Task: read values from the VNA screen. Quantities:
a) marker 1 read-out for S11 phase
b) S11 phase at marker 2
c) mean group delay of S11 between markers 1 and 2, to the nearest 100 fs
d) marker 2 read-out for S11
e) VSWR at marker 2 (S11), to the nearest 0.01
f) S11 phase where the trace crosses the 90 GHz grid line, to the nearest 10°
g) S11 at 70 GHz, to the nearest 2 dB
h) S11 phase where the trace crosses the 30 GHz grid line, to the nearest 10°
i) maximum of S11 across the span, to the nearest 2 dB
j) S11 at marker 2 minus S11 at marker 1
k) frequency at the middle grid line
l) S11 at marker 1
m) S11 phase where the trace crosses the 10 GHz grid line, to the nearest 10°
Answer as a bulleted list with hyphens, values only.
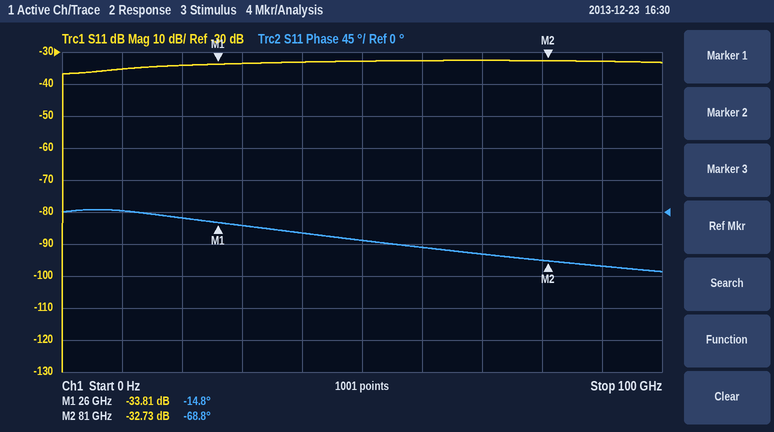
- -14.8°
- -68.8°
- 2.7 ps
- -32.73 dB
- 1.05
- -80°
- -32 dB
- -20°
- -32 dB
- 1.08 dB
- 50 GHz
- -33.81 dB
- 0°
